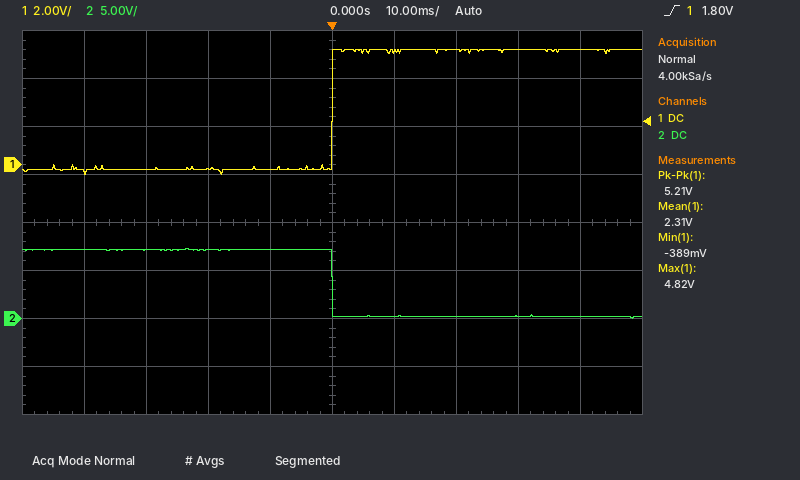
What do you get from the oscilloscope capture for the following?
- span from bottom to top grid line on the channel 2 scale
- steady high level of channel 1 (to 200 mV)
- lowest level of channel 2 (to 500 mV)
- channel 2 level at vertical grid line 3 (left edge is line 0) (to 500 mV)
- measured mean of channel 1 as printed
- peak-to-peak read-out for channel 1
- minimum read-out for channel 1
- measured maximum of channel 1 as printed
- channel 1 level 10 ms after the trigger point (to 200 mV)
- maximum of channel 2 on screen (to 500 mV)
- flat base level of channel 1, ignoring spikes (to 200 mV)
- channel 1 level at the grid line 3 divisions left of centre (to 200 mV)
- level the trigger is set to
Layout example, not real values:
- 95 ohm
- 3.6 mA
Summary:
- 40 V
- 4.8 V
- 0.0 V
- 7.0 V
- 2.31 V
- 5.21 V
- -389 mV
- 4.82 V
- 4.8 V
- 7.5 V
- -200 mV
- -200 mV
- 1.80 V
